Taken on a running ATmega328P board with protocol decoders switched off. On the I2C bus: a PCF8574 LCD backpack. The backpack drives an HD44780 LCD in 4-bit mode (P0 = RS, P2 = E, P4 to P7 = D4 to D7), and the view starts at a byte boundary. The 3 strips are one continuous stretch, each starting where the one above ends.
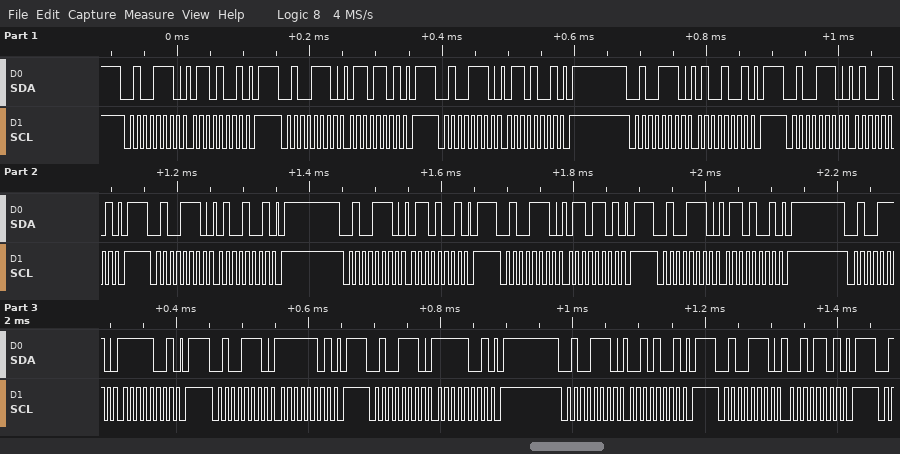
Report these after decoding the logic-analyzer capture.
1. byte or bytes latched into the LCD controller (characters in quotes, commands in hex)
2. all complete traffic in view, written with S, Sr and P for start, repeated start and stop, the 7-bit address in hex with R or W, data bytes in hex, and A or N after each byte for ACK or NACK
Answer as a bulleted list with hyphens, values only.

- 'd' 'o'
- S 27W A 69 A P S 27W A 6D A P S 27W A 69 A P S 27W A 49 A P S 27W A 4D A P S 27W A 49 A P S 27W A 69 A P S 27W A 6D A P S 27W A 69 A P S 27W A F9 A P S 27W A FD A P S 27W A F9 A P S 27W A 29 A P S 27W A 2D A P
